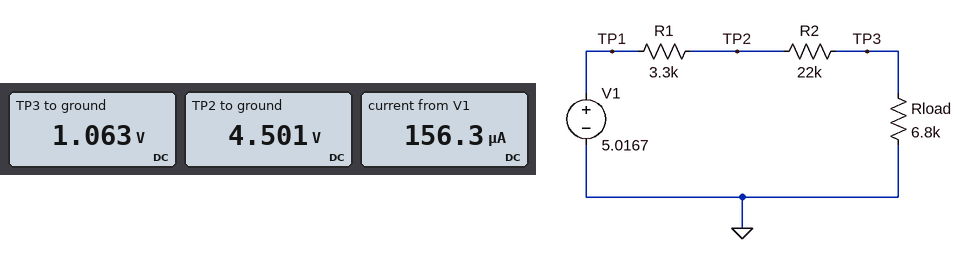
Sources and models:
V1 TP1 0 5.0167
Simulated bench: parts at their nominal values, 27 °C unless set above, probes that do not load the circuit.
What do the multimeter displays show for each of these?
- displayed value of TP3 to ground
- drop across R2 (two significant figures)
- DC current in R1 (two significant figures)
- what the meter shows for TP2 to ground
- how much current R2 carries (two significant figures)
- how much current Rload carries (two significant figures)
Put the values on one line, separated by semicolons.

1.063 V; 3.4 V; 160 µA; 4.501 V; 160 µA; 160 µA
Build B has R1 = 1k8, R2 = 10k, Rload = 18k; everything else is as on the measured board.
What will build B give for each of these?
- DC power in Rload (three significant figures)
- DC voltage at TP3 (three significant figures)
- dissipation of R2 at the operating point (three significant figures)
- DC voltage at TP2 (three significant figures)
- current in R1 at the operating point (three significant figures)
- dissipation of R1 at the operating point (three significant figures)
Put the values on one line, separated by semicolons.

510 µW; 3.03 V; 283 µW; 4.71 V; 168 µA; 51.0 µW
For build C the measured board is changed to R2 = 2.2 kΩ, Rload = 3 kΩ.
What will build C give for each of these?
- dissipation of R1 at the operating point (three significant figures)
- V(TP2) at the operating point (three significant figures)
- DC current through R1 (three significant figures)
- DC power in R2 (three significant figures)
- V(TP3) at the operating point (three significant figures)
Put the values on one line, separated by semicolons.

1.15 mW; 3.07 V; 590 µA; 766 µW; 1.77 V
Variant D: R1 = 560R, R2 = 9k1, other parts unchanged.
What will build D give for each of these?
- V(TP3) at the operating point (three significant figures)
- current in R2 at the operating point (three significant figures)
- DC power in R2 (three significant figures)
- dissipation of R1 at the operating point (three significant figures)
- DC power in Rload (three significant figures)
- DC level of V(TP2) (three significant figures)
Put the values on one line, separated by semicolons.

2.07 V; 305 µA; 845 µW; 52.0 µW; 632 µW; 4.85 V
